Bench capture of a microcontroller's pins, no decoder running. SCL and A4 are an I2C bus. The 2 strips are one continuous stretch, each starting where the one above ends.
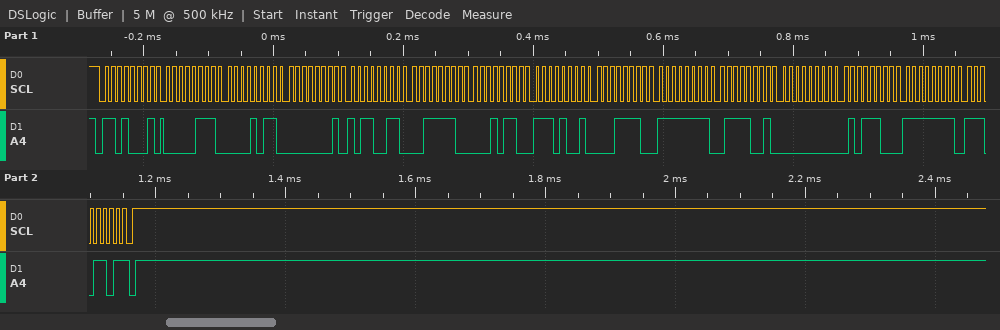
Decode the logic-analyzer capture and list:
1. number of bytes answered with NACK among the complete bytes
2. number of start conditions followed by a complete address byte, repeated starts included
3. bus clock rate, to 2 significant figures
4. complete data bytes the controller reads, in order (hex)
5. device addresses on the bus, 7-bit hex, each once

1
1
100 kHz
07 0B 01 B3 3E 16 E9 1E FF 79 00 5C FF ED
0x68
